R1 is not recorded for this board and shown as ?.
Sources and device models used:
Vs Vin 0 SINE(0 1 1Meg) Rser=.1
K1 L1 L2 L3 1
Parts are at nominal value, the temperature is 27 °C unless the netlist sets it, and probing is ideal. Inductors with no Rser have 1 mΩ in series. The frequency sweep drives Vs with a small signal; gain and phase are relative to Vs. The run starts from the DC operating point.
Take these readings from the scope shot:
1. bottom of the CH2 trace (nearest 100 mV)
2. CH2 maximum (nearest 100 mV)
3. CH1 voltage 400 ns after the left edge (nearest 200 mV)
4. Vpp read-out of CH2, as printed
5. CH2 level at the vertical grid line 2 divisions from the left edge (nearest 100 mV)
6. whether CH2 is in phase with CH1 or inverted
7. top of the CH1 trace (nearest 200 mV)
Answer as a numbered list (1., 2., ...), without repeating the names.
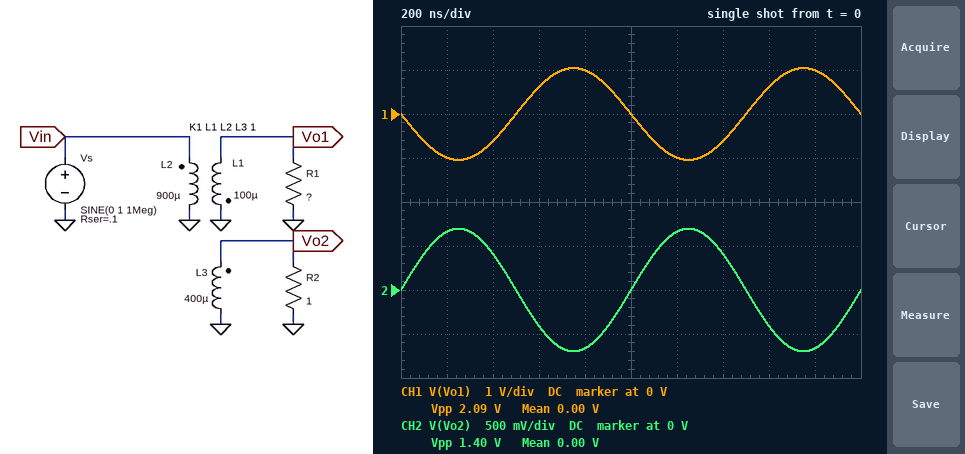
1. -700 mV
2. 700 mV
3. -600 mV
4. 1.40 V
5. 400 mV
6. inverted
7. 1.0 V
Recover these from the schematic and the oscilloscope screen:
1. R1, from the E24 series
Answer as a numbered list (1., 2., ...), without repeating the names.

1. 0.62 Ω
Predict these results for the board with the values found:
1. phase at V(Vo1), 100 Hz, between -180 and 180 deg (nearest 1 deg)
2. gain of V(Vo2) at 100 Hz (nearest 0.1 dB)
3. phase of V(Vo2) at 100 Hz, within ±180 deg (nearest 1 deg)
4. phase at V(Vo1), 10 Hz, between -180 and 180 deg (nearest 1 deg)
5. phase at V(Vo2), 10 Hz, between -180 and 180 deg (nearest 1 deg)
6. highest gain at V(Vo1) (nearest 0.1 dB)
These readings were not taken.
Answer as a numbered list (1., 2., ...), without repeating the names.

1. -151 deg
2. -4.3 dB
3. 29 deg
4. -100 deg
5. 80 deg
6. 0.4 dB
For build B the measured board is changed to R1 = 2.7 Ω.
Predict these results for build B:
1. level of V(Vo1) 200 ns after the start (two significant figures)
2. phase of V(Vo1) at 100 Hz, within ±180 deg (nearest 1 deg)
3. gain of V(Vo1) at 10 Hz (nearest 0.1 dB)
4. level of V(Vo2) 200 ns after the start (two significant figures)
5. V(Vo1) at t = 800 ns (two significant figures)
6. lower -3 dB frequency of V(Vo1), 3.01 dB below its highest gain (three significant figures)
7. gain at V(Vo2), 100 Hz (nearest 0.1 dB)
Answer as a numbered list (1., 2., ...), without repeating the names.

1. -1.6 V
2. -137 deg
3. -14.6 dB
4. 1.1 V
5. 1.6 V
6. 92.4 Hz
7. -1.5 dB
